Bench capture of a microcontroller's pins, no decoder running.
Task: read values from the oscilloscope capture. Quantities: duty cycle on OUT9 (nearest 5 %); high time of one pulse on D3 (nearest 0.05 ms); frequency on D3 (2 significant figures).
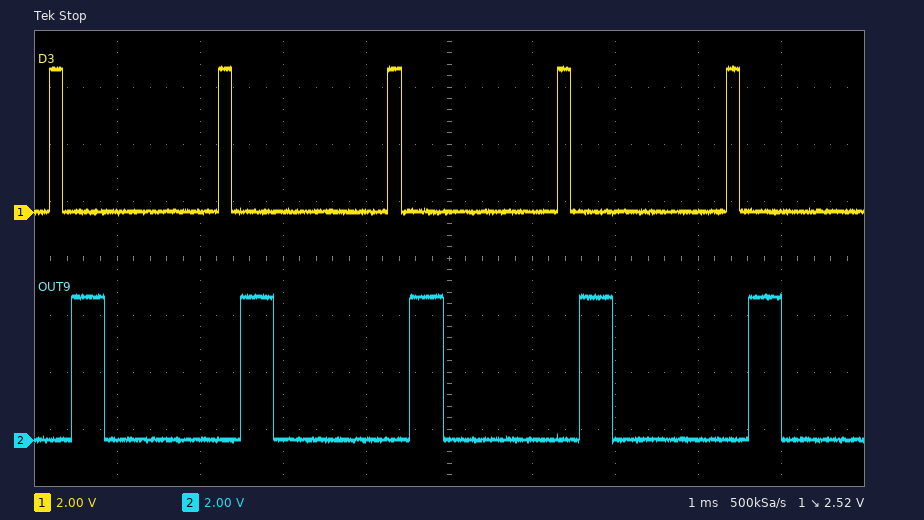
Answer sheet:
20 %
0.15 ms
490 Hz
